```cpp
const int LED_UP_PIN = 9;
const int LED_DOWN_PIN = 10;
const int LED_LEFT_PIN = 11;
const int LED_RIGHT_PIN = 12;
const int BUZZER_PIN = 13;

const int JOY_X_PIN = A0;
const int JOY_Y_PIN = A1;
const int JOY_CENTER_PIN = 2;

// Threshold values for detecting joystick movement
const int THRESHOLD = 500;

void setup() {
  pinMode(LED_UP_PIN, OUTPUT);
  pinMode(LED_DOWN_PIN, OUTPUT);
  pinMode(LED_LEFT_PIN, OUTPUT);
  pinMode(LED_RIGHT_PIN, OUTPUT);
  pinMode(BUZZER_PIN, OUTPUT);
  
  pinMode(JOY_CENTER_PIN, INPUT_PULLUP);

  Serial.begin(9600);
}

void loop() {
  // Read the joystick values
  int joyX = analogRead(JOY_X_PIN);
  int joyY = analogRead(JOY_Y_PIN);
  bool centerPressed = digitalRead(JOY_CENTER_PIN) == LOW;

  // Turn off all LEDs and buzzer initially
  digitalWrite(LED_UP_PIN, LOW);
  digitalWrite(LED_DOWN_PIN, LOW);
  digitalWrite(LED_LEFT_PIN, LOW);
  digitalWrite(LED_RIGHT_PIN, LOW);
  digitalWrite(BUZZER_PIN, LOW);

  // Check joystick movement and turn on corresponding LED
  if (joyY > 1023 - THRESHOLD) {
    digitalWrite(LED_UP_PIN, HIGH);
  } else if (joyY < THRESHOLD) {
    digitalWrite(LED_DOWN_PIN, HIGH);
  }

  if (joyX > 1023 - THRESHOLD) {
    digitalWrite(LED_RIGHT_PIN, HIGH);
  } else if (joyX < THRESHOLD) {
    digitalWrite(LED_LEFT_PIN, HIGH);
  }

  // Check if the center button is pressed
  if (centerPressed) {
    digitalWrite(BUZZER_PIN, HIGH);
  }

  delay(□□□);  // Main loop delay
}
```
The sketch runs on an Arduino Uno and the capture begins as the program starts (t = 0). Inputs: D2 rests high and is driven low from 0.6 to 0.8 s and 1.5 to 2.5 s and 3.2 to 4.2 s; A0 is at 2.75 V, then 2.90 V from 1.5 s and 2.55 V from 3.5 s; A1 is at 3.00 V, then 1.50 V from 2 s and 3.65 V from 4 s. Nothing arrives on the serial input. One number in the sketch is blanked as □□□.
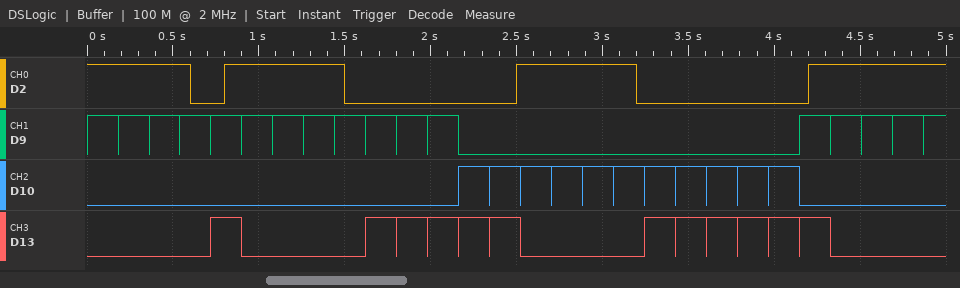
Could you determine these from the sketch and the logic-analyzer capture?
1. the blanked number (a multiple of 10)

180
